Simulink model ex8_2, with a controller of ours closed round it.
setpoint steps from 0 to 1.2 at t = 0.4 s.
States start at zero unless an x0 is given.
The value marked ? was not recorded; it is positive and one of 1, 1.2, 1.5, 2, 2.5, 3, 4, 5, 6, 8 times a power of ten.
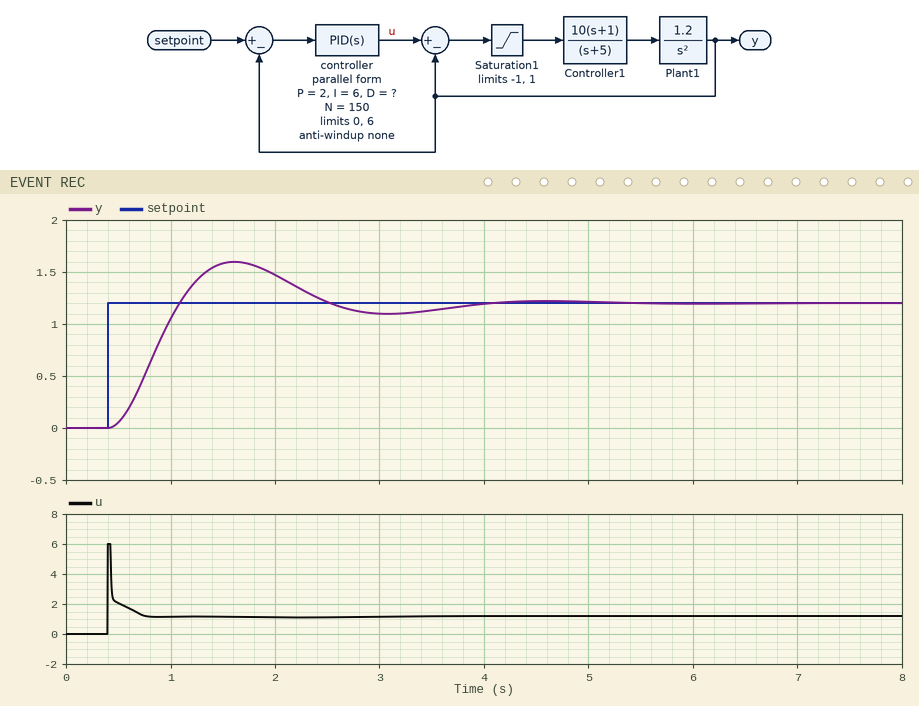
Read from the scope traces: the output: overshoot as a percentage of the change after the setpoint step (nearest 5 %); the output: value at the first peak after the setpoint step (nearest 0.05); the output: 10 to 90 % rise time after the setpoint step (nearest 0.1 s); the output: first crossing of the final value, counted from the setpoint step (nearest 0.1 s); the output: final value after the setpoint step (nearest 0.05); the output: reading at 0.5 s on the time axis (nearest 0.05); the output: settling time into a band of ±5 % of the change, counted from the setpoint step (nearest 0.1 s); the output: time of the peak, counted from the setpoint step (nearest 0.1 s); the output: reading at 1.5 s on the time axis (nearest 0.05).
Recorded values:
35 %
1.60
0.5 s
0.7 s
1.20
0.05
3.2 s
1.2 s
1.60
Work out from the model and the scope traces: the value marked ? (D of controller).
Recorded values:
1
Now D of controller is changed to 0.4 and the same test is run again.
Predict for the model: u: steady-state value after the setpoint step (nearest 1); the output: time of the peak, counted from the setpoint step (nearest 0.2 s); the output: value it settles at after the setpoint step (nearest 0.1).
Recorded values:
1
1.0 s
1.2
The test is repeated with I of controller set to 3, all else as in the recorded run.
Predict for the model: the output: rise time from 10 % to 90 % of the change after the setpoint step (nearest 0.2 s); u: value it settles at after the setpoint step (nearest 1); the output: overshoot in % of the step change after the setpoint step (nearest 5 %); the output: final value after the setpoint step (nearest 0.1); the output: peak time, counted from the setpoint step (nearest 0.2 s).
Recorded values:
0.6 s
1
15 %
1.2
1.6 s
